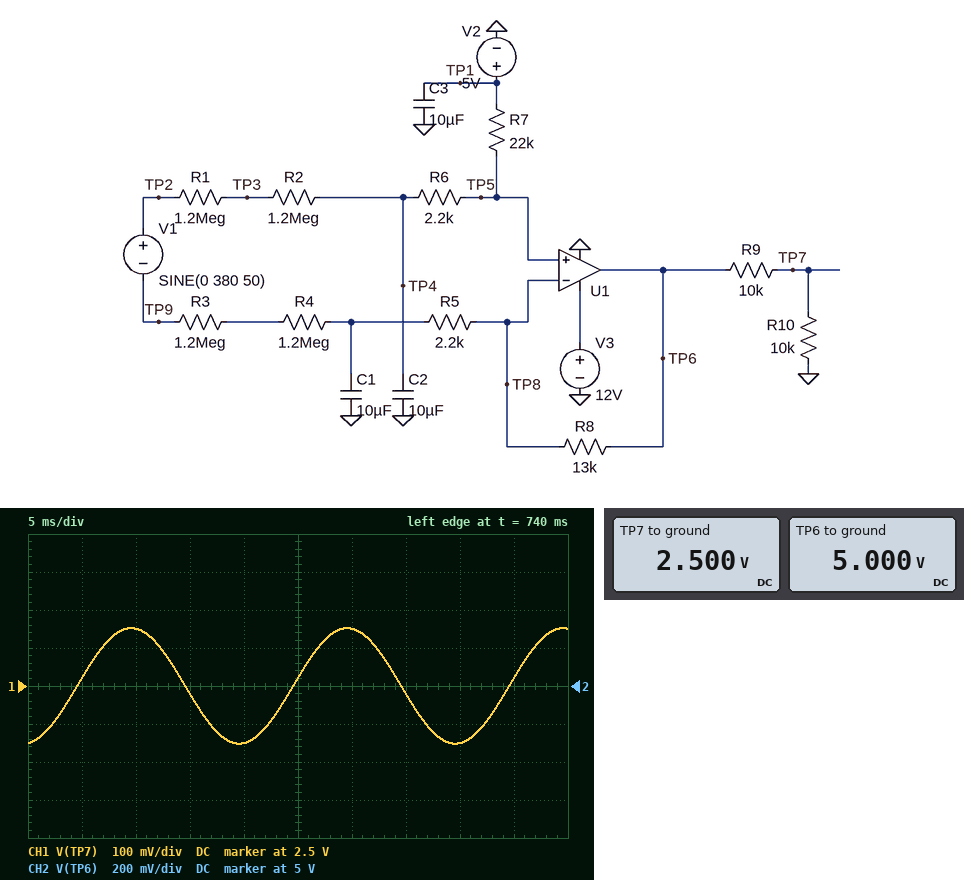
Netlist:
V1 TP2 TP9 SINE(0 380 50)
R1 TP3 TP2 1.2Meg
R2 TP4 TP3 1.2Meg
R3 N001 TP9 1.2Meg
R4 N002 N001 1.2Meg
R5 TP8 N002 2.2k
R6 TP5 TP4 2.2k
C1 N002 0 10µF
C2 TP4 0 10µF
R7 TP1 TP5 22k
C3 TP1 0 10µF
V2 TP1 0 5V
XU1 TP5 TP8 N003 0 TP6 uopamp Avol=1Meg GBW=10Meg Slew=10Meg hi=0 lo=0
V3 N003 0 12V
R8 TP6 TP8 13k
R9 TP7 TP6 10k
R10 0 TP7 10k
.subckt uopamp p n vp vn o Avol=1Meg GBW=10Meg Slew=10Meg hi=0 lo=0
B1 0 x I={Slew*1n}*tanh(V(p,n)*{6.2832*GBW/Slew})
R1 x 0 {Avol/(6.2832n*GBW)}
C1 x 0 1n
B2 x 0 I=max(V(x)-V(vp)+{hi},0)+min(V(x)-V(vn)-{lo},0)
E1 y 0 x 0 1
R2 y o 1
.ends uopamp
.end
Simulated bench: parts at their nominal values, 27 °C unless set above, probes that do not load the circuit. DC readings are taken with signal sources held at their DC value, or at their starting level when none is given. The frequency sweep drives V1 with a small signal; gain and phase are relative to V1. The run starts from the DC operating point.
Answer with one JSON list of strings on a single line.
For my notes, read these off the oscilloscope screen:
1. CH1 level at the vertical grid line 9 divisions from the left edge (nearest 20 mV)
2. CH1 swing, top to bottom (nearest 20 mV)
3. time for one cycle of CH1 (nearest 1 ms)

["2.52 V", "300 mV", "20 ms"]
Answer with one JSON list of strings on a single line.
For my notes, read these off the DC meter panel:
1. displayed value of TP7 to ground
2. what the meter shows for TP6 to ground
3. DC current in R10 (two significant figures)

["2.500 V", "5.000 V", "250 µA"]
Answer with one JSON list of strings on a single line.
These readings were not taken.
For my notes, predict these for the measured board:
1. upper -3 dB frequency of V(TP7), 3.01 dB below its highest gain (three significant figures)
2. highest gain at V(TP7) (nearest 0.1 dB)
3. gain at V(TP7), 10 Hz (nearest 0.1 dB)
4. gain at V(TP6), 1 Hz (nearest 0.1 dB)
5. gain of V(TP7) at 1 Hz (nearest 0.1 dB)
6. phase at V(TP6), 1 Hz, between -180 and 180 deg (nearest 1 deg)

["3.29 Hz", "-48.8 dB", "-55.7 dB", "-44.3 dB", "-50.3 dB", "-15 deg"]
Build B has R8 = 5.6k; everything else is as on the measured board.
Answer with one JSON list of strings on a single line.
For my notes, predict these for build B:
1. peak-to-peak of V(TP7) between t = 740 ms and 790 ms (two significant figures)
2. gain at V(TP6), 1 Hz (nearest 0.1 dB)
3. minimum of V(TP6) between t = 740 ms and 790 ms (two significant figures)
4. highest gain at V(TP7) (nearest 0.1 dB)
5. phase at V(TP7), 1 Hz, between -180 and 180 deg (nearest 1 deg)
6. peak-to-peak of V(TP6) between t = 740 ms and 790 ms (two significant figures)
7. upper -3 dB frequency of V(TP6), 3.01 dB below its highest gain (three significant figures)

["140 mV", "-48.4 dB", "4.9 V", "-50.8 dB", "-30 deg", "290 mV", "850 mHz"]
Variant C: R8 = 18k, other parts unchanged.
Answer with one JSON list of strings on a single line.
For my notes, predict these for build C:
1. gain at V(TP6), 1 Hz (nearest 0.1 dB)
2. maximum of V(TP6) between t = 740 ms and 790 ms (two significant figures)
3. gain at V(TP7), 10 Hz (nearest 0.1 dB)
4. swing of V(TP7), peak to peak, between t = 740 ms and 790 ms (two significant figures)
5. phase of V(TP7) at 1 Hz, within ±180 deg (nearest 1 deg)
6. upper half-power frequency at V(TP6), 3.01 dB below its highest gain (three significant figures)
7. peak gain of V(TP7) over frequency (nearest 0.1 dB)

["-42.2 dB", "5.4 V", "-53.1 dB", "410 mV", "-10 deg", "5.87 Hz", "-47.6 dB"]
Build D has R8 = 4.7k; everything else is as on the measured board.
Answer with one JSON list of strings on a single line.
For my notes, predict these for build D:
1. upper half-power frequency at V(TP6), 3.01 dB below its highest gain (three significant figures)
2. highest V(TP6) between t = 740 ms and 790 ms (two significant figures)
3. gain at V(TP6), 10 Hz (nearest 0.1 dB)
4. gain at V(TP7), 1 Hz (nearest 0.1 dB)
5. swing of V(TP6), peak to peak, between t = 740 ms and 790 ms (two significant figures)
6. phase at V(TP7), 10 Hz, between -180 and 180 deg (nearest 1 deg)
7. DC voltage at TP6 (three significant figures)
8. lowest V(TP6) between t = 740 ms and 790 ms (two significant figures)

["796 mHz", "5.1 V", "-57.4 dB", "-55.0 dB", "250 mV", "-59 deg", "5.00 V", "4.9 V"]
